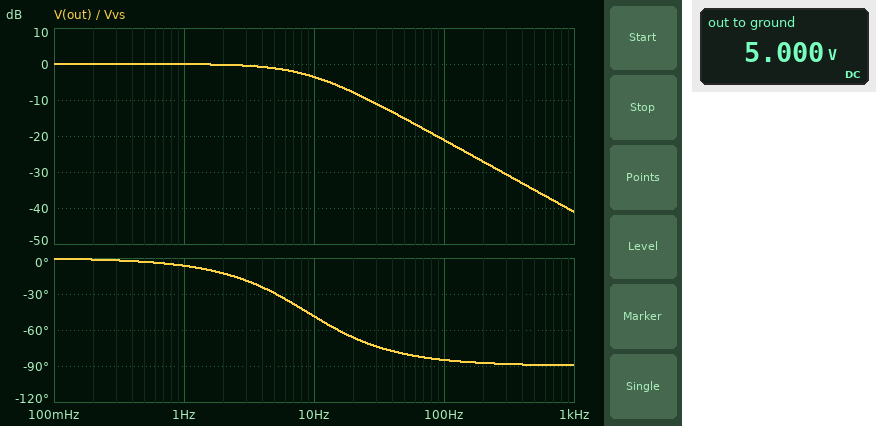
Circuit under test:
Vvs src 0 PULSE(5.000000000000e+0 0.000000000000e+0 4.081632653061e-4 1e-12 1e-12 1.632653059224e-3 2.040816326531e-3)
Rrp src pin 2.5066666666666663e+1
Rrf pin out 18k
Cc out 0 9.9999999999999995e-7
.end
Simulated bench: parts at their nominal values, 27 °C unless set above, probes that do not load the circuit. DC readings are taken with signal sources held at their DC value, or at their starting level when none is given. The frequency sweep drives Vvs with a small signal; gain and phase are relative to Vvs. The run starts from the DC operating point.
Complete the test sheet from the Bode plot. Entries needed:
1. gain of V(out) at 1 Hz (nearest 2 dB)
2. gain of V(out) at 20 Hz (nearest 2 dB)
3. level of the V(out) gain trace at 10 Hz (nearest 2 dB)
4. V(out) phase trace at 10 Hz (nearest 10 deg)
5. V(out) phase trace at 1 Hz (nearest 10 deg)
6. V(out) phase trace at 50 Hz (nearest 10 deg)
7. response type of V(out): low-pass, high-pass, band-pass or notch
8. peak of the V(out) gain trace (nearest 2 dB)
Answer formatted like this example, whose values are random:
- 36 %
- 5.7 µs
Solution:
- 0 dB
- -8 dB
- -4 dB
- -50 deg
- -10 deg
- -80 deg
- low-pass
- 0 dB
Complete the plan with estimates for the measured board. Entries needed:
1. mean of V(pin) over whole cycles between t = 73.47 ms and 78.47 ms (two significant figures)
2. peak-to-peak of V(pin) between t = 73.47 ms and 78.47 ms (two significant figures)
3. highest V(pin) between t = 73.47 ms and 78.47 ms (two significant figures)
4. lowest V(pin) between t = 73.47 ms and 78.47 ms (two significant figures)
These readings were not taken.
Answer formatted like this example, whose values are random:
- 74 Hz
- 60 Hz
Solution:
- 1.0 V
- 5.0 V
- 5.0 V
- 1.4 mV
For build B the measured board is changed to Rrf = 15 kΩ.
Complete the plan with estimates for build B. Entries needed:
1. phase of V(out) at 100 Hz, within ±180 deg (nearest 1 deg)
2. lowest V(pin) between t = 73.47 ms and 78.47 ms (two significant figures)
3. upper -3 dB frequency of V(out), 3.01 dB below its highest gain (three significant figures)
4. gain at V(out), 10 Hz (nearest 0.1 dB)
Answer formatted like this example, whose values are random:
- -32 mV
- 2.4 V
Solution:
- -84 deg
- 1.6 mV
- 10.6 Hz
- -2.8 dB
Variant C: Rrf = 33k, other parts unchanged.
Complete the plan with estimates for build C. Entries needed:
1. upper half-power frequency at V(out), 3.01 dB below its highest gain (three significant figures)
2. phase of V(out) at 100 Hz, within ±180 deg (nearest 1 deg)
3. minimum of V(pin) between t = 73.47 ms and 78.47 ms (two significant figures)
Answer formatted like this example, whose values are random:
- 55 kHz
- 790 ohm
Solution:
- 4.82 Hz
- -87 deg
- 1.0 mV
